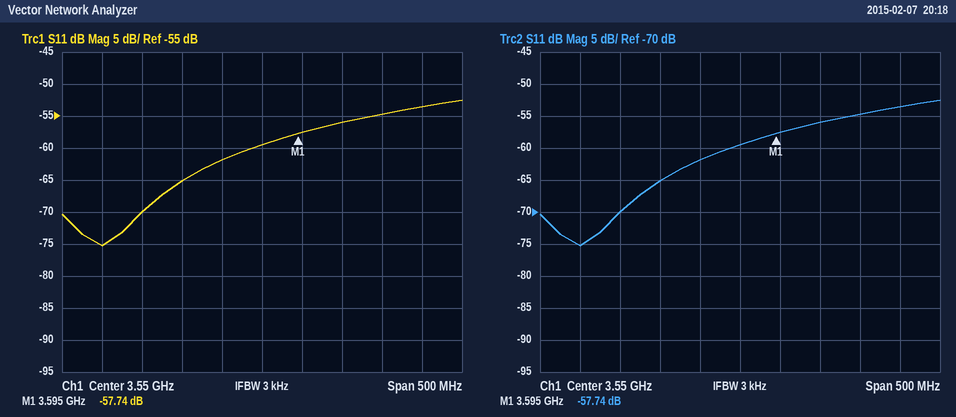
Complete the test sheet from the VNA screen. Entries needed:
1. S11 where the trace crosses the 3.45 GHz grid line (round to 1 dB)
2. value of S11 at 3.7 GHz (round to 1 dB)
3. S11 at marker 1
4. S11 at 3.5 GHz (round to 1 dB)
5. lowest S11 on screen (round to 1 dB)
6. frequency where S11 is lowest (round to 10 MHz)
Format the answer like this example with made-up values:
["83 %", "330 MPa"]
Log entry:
["-65 dB", "-55 dB", "-57.74 dB", "-62 dB", "-75 dB", "3.35 GHz"]
